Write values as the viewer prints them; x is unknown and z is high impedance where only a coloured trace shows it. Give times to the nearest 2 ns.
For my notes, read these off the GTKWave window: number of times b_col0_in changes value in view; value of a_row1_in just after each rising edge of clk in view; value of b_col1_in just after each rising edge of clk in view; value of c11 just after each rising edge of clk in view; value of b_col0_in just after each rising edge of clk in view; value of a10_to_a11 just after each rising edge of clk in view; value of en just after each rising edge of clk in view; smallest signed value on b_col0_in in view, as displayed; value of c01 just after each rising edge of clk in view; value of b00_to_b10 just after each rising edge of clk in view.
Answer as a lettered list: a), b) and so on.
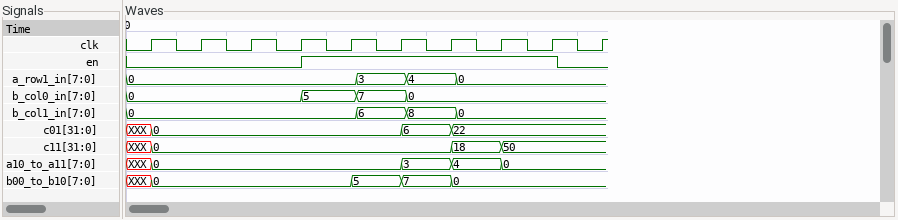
a) 3
b) 0, 0, 0, 0, 0, 3, 4, 0, 0, 0
c) 0, 0, 0, 0, 0, 6, 8, 0, 0, 0
d) 0, 0, 0, 0, 0, 0, 18, 50, 50, 50
e) 0, 0, 0, 5, 5, 7, 0, 0, 0, 0
f) 0, 0, 0, 0, 0, 3, 4, 0, 0, 0
g) 0 0 0 1 1 1 1 1 1 0
h) 0
i) 0, 0, 0, 0, 0, 6, 22, 22, 22, 22
j) 0, 0, 0, 0, 5, 7, 0, 0, 0, 0
